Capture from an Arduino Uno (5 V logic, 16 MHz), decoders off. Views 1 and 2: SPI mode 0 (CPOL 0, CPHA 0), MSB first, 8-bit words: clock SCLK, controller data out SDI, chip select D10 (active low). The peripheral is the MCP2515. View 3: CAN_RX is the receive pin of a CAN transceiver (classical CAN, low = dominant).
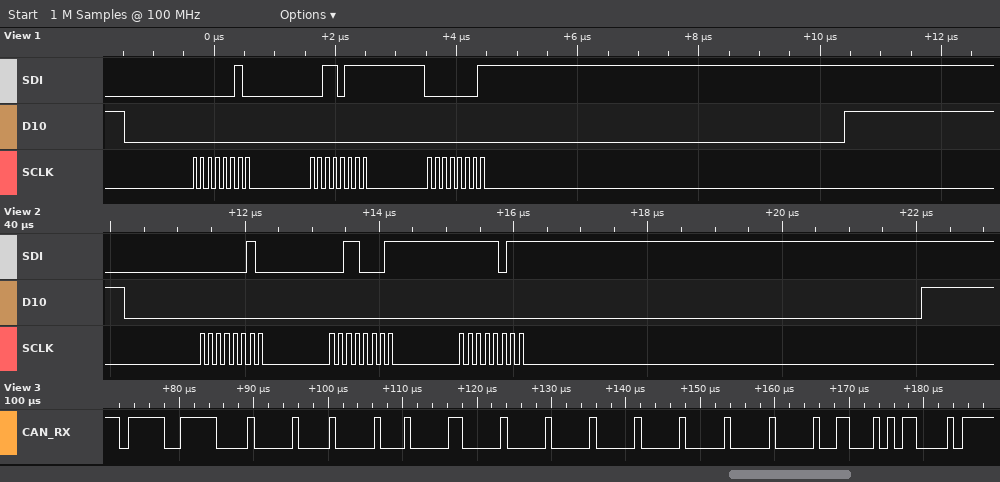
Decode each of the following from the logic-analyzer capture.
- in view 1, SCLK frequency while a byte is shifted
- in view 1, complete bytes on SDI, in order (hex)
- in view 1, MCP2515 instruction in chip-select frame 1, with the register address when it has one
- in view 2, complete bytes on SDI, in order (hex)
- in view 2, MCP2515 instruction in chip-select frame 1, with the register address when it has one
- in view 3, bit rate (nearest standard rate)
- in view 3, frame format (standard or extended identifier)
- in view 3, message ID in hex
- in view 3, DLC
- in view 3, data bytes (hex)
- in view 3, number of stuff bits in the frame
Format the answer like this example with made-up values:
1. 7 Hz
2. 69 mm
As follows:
1. 8 MHz
2. 0x02 0x37 0x01
3. WRITE 0x37
4. 02 31 FB
5. WRITE 0x31
6. 1000 kbit/s
7. standard
8. 0x7DF
9. 8
10. 02 01 04 00 00 00 00 00
11. 13
